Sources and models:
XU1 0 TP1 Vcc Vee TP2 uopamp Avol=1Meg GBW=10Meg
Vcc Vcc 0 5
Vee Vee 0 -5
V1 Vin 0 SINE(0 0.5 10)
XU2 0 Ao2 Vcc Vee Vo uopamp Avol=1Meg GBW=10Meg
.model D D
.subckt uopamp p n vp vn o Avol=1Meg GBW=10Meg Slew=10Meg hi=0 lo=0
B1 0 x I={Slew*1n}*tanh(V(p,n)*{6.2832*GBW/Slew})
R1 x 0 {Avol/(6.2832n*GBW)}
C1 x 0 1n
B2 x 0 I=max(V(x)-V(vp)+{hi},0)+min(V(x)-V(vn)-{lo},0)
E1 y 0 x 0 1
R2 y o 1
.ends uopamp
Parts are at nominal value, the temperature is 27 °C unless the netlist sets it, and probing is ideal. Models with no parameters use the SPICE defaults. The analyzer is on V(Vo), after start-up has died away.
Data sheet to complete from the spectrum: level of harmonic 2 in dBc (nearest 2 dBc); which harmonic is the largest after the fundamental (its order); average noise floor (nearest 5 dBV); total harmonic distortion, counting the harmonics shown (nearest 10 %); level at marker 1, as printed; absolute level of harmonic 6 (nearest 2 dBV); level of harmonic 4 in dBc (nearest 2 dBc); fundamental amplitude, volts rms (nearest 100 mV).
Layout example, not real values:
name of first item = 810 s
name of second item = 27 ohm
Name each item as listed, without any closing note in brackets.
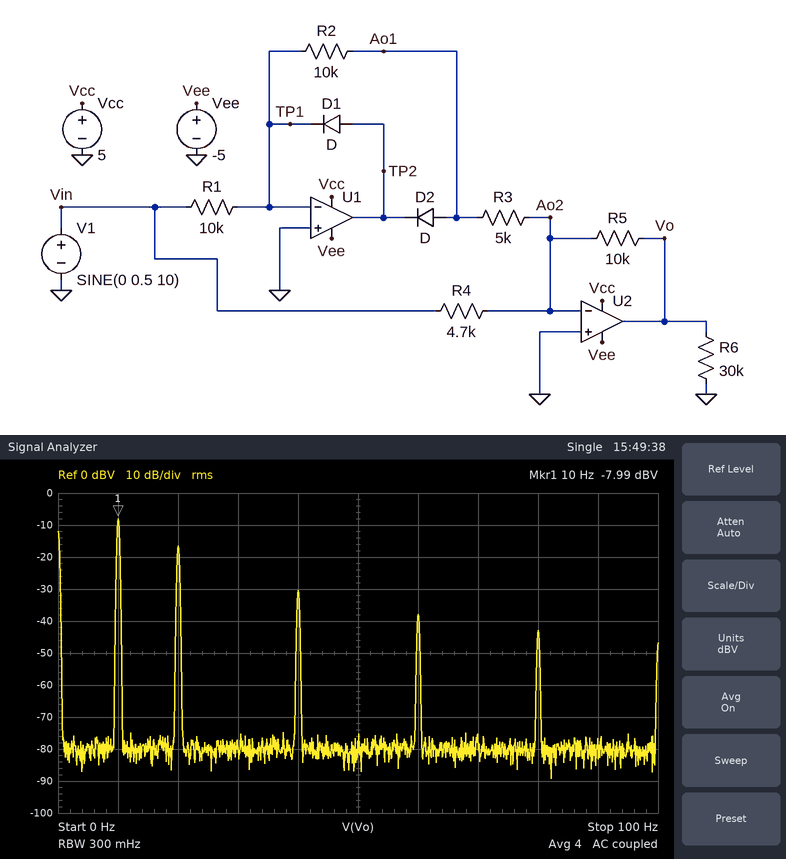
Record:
level of harmonic 2 in dBc = -8 dBc
which harmonic is the largest after the fundamental = 2
average noise floor = -80 dBV
total harmonic distortion, counting the harmonics shown = 40 %
level at marker 1, as printed = -7.99 dBV
absolute level of harmonic 6 = -38 dBV
level of harmonic 4 in dBc = -22 dBc
fundamental amplitude, volts rms = 400 mV
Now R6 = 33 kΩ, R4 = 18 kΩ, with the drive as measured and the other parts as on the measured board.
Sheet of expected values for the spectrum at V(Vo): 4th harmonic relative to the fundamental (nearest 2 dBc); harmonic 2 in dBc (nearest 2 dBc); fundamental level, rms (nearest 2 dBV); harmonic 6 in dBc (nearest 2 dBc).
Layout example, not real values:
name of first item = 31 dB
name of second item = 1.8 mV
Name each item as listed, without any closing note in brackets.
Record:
4th harmonic relative to the fundamental = -14 dBc
harmonic 2 in dBc = 0 dBc
fundamental level, rms = -16 dBV
harmonic 6 in dBc = -22 dBc
